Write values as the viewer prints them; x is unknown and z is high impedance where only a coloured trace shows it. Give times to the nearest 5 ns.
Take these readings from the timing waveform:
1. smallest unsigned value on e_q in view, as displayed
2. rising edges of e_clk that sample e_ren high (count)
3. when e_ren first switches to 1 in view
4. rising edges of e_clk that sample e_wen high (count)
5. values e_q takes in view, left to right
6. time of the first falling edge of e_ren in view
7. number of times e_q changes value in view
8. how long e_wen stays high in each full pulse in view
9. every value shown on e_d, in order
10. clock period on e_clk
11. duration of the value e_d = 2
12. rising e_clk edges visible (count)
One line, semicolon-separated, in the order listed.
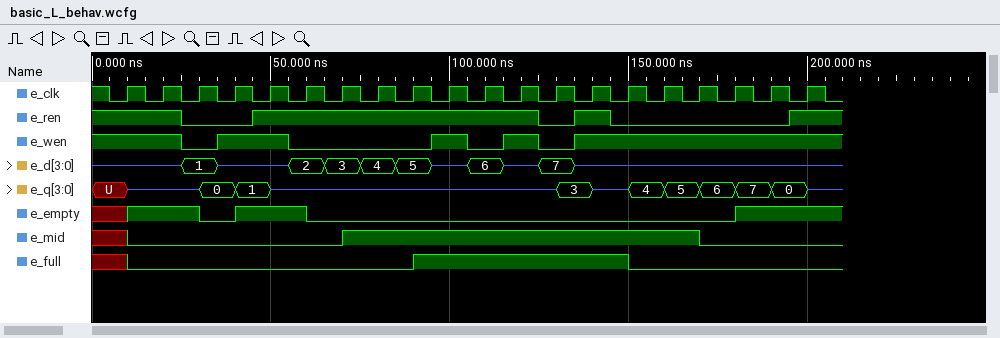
0; 12; 45 ns; 13; U, z, 0, 1, z, 3, z, 4, 5, 6, 7, 0, z; 25 ns; 12; 20 ns, 10 ns, 10 ns; z, 1, z, 2, 3, 4, 5, z, 6, z, 7, z; 10 ns; 10 ns; 20
